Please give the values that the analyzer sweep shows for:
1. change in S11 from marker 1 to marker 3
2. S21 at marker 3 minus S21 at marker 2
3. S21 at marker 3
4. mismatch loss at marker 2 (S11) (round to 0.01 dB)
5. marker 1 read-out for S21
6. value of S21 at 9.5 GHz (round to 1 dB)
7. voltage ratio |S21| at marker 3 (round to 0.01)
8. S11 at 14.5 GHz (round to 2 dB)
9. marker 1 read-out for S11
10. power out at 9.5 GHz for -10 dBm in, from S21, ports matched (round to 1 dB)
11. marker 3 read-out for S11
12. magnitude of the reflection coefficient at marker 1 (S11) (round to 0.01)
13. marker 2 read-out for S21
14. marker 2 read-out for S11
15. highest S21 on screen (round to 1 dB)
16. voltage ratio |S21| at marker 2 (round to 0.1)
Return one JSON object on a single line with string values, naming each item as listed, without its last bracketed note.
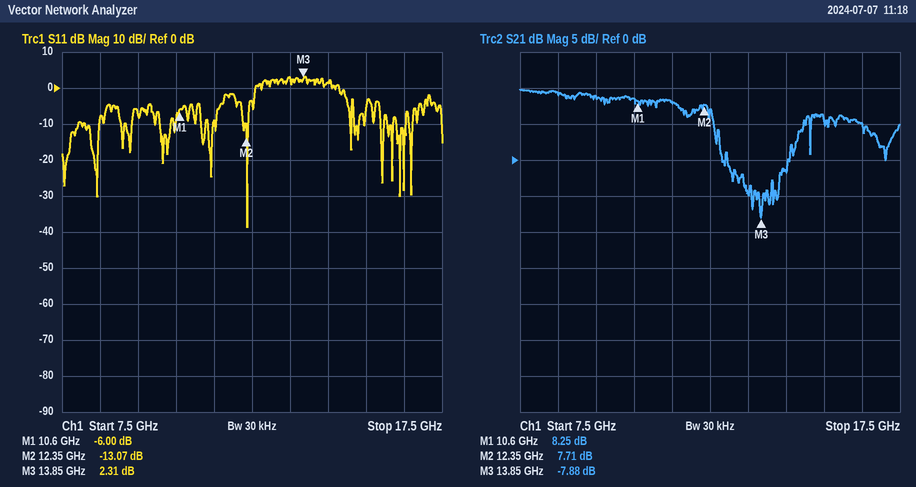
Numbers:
{"change in S11 from marker 1 to marker 3": "8.31 dB", "S21 at marker 3 minus S21 at marker 2": "-15.59 dB", "S21 at marker 3": "-7.88 dB", "mismatch loss at marker 2 (S11)": "0.22 dB", "marker 1 read-out for S21": "8.25 dB", "value of S21 at 9.5 GHz": "9 dB", "voltage ratio |S21| at marker 3": "0.40", "S11 at 14.5 GHz": "2 dB", "marker 1 read-out for S11": "-6.00 dB", "power out at 9.5 GHz for -10 dBm in, from S21, ports matched": "-1 dBm", "marker 3 read-out for S11": "2.31 dB", "magnitude of the reflection coefficient at marker 1 (S11)": "0.50", "marker 2 read-out for S21": "7.71 dB", "marker 2 read-out for S11": "-13.07 dB", "highest S21 on screen": "10 dB", "voltage ratio |S21| at marker 2": "2.4"}
